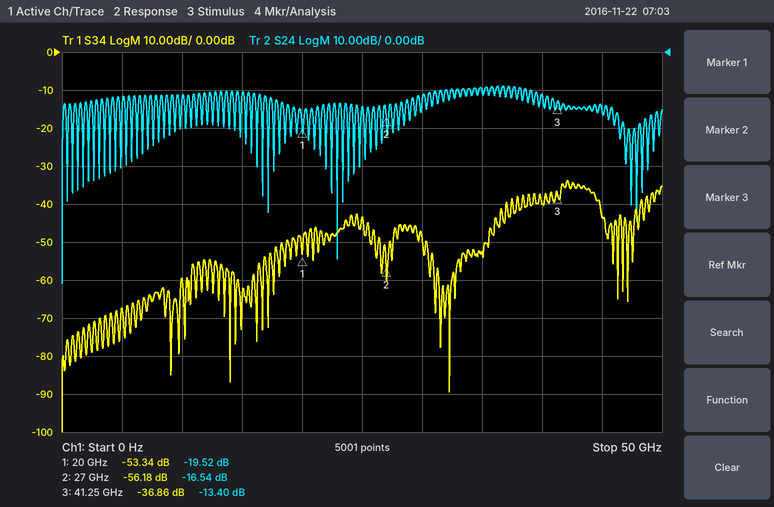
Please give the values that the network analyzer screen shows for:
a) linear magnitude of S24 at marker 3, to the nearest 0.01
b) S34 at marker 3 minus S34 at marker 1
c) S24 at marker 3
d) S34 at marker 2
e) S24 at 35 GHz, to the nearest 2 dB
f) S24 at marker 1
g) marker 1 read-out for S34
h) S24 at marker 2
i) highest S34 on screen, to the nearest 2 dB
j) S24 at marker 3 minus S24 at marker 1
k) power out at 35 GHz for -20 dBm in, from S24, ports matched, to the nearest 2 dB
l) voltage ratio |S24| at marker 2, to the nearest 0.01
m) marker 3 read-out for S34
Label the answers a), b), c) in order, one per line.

a) 0.21
b) 16.48 dB
c) -13.40 dB
d) -56.18 dB
e) -10 dB
f) -19.52 dB
g) -53.34 dB
h) -16.54 dB
i) -34 dB
j) 6.12 dB
k) -30 dBm
l) 0.15
m) -36.86 dB
